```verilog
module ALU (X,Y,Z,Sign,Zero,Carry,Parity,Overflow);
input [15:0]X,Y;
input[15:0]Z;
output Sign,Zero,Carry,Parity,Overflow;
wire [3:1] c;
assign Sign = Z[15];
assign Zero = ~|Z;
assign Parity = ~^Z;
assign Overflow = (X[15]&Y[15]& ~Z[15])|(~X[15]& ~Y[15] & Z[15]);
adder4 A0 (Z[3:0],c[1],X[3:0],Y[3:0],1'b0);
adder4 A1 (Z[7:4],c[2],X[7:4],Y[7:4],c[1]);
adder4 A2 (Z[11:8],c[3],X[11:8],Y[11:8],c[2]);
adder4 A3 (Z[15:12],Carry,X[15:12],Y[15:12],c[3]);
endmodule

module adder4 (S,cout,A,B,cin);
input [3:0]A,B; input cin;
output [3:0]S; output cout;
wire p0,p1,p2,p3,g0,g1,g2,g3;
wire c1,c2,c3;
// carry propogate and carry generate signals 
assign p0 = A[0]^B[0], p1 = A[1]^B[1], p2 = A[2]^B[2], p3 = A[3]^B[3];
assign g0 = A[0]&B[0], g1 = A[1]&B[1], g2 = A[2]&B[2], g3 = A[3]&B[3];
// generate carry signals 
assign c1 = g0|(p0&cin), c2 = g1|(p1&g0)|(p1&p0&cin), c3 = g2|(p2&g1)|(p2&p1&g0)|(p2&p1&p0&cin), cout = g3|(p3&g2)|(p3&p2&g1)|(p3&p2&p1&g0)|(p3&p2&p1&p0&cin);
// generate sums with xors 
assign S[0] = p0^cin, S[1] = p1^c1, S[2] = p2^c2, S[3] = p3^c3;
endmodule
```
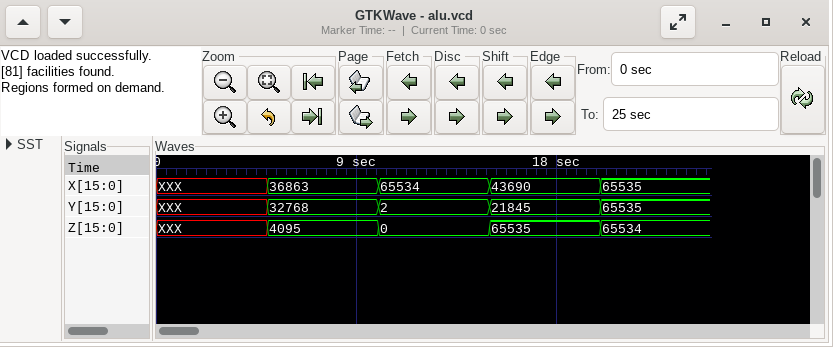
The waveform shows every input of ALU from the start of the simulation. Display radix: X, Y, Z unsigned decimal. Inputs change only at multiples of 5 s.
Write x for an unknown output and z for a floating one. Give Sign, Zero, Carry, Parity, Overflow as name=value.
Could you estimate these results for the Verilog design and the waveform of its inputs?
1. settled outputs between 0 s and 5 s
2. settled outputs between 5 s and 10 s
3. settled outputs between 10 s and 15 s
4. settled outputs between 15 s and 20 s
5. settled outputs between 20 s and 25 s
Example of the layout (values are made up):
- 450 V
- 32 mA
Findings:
- Sign=x, Zero=x, Carry=x, Parity=x, Overflow=x
- Sign=0, Zero=0, Carry=1, Parity=1, Overflow=1
- Sign=0, Zero=1, Carry=1, Parity=1, Overflow=0
- Sign=1, Zero=0, Carry=0, Parity=1, Overflow=0
- Sign=1, Zero=0, Carry=1, Parity=0, Overflow=0
